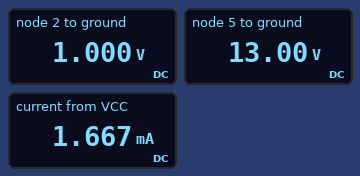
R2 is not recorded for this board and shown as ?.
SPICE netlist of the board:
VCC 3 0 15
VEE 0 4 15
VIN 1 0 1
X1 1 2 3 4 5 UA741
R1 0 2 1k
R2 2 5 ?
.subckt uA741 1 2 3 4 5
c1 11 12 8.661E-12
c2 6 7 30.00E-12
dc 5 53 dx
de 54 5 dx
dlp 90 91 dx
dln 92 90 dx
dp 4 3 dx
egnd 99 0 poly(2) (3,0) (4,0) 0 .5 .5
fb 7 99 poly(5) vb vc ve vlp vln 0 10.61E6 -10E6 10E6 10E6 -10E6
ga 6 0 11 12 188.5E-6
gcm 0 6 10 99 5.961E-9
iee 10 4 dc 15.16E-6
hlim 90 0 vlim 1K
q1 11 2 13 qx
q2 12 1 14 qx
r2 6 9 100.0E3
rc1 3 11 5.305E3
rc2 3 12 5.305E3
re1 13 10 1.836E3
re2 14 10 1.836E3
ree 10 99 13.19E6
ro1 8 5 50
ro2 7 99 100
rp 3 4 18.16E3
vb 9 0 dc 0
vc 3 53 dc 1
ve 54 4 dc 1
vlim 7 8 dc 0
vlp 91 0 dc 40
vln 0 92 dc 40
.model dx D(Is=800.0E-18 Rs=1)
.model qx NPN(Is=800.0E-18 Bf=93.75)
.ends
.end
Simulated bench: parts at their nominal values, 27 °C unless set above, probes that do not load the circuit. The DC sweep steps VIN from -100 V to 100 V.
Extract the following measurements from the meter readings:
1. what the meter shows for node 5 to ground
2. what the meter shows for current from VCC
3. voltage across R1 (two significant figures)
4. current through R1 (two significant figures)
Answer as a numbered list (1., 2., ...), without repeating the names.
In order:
1. 13.00 V
2. 1.667 mA
3. 1.0 V
4. 1.0 mA
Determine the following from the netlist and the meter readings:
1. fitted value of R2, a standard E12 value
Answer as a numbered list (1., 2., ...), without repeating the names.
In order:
1. 12 kΩ
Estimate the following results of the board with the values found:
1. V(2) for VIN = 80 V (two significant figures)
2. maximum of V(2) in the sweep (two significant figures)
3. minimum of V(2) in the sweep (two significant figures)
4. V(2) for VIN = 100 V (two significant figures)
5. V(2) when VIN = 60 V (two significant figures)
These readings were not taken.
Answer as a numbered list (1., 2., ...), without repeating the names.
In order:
1. -1.1 V
2. 1.1 V
3. -1.1 V
4. -1.1 V
5. -1.1 V
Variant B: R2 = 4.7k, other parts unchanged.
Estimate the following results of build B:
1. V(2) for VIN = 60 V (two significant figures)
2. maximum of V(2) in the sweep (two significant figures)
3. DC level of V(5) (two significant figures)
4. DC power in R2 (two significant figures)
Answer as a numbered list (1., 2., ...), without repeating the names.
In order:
1. -2.6 V
2. 2.6 V
3. 5.7 V
4. 4.7 mW
